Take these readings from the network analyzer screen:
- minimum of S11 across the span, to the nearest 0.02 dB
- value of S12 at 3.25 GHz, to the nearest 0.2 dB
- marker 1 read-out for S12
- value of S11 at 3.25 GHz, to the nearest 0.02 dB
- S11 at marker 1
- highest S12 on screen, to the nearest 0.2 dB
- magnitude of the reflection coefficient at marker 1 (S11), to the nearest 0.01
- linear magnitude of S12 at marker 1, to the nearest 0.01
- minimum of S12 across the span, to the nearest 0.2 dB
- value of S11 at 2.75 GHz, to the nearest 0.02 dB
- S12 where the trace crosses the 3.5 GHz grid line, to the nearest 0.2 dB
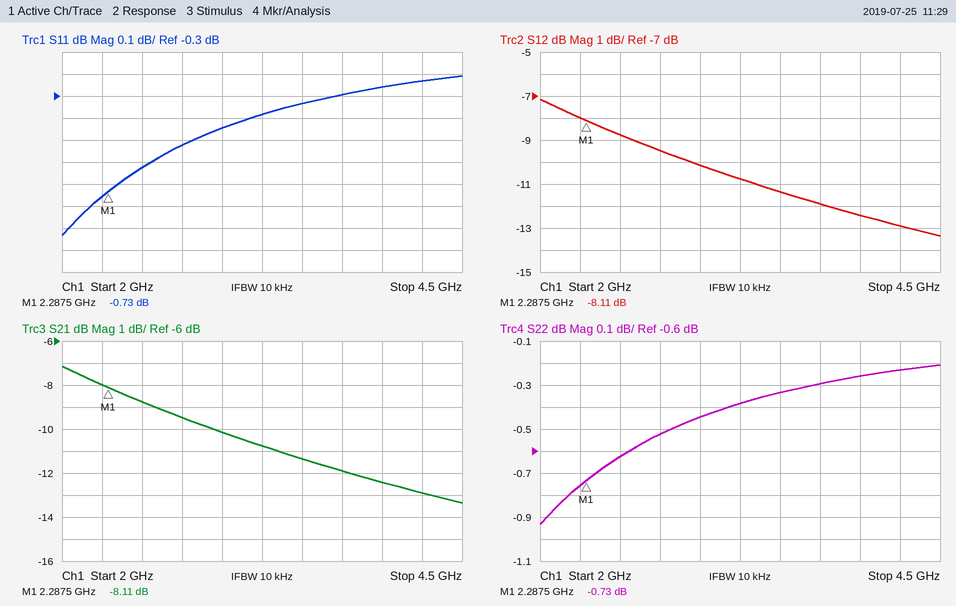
-0.94 dB
-10.8 dB
-8.11 dB
-0.38 dB
-0.73 dB
-7.2 dB
0.92
0.39
-13.4 dB
-0.52 dB
-11.4 dB
